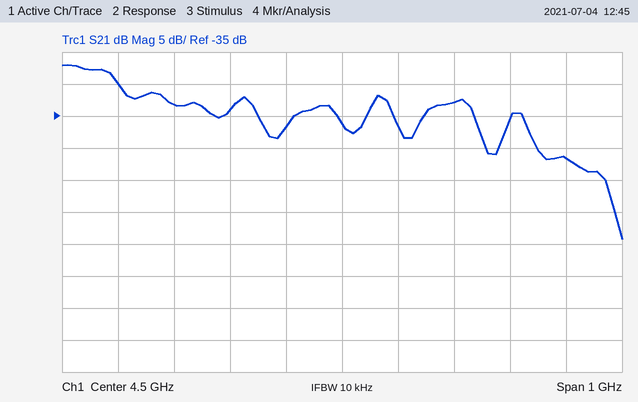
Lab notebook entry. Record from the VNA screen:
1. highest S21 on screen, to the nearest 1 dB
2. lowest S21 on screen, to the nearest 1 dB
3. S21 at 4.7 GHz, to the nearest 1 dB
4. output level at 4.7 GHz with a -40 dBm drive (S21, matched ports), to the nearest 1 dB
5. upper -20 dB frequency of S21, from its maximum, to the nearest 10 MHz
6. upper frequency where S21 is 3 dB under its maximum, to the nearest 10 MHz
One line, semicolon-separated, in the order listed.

-27 dB; -54 dB; -33 dB; -73 dBm; 4.98 GHz; 4.10 GHz
